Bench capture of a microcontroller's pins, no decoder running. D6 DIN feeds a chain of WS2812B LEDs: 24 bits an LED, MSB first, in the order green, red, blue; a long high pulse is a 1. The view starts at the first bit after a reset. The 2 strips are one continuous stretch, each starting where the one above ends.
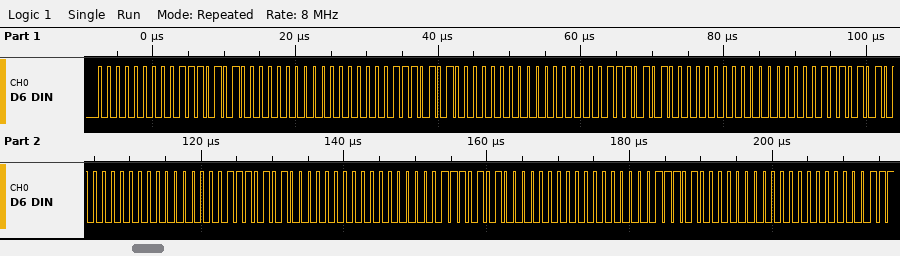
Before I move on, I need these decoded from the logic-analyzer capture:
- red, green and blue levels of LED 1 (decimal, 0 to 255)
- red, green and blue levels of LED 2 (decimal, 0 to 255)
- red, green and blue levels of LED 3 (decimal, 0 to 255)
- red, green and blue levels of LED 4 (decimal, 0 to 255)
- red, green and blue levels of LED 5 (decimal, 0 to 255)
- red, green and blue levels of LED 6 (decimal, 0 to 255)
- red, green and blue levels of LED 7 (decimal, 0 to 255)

117, 0, 0
117, 0, 0
117, 0, 0
117, 0, 0
117, 0, 0
117, 0, 0
116, 0, 0
